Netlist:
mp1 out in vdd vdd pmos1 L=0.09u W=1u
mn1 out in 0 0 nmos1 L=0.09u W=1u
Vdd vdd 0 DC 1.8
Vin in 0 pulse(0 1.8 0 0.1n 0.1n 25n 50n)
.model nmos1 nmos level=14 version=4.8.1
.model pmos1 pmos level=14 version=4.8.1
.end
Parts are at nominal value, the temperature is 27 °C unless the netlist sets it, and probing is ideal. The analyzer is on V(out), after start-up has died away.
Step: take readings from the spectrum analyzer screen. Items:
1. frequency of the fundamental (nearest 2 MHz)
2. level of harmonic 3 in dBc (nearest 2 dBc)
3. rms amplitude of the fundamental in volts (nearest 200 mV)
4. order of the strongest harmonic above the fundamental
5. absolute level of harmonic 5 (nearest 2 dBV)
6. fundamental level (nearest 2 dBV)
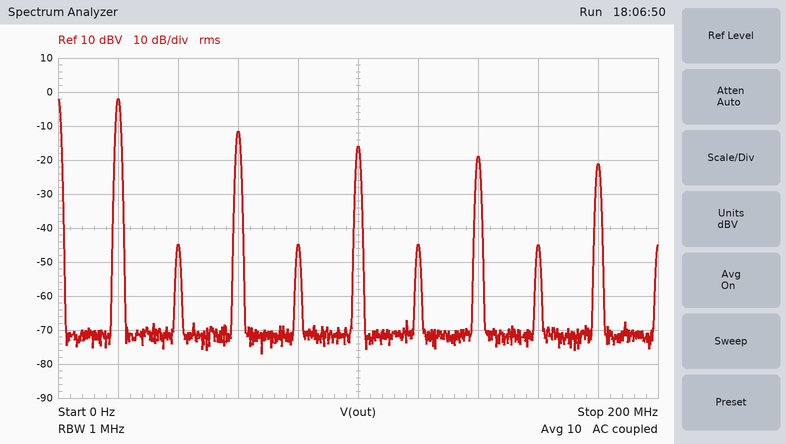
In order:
20 MHz
-10 dBc
800 mV
3
-16 dBV
-2 dBV
